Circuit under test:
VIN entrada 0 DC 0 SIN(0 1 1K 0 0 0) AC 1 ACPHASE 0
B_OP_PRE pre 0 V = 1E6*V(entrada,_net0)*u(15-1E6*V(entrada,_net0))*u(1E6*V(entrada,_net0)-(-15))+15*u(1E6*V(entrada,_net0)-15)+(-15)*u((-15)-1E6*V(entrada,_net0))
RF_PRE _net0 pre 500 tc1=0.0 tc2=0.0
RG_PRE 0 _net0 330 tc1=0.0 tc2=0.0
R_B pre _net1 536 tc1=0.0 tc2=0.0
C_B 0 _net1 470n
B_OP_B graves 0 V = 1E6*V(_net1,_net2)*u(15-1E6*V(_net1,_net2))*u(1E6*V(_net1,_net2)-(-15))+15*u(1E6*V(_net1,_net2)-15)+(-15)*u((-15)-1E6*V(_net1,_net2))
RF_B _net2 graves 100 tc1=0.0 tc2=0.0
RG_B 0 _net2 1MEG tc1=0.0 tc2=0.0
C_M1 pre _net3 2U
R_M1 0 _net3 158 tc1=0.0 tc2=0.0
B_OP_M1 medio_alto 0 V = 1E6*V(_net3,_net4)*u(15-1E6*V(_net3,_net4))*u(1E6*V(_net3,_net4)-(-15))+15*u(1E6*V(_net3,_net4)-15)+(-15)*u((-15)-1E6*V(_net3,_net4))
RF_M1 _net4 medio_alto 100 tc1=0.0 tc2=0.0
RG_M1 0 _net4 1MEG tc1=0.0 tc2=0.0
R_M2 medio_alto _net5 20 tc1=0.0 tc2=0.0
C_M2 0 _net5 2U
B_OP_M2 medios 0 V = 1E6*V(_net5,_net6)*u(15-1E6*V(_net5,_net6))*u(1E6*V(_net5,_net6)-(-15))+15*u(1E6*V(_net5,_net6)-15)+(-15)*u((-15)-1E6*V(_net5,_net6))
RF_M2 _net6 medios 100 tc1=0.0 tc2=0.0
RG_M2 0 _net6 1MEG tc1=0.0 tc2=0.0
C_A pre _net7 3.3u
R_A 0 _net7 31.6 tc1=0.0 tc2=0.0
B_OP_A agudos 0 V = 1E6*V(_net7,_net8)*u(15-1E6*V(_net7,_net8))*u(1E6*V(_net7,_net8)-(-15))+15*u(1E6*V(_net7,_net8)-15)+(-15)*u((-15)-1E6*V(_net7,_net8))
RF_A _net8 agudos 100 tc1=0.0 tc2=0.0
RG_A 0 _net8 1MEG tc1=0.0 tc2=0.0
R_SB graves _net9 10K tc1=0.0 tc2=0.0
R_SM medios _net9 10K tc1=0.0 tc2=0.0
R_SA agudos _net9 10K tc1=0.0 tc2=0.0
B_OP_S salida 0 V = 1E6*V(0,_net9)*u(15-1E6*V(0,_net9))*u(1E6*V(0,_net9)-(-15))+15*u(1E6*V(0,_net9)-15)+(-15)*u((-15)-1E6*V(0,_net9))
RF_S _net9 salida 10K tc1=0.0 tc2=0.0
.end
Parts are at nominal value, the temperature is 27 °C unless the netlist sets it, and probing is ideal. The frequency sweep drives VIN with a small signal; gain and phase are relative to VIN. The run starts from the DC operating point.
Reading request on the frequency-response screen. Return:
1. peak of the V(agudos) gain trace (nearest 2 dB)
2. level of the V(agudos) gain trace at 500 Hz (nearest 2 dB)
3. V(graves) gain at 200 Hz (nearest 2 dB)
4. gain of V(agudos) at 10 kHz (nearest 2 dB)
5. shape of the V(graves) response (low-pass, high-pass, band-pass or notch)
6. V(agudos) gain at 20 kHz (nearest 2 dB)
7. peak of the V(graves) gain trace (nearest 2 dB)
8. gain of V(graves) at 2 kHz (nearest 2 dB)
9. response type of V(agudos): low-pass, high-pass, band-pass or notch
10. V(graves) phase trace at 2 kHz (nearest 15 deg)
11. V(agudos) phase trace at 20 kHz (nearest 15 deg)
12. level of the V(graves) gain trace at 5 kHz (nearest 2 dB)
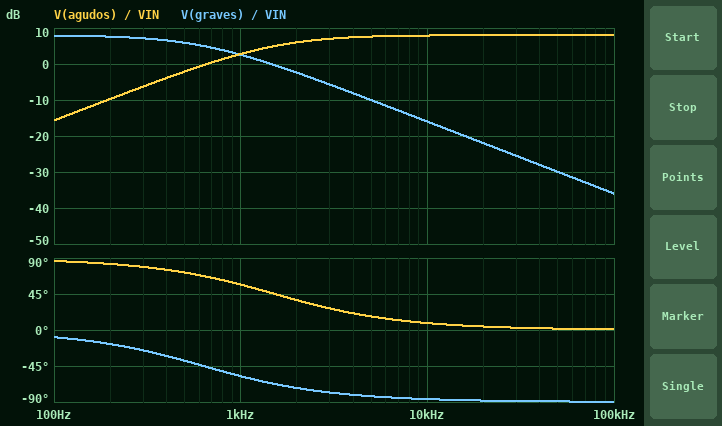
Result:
8 dB
-2 dB
8 dB
8 dB
low-pass
8 dB
8 dB
-2 dB
high-pass
-75 deg
0 deg
-10 dB
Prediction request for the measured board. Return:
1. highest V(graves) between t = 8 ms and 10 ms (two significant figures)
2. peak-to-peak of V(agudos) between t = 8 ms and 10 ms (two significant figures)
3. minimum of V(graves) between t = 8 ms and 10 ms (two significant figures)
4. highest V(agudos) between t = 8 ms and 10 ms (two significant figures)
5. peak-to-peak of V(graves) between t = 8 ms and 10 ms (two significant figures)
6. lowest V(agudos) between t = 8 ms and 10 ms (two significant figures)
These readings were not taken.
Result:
1.3 V
2.8 V
-1.3 V
1.4 V
2.7 V
-1.4 V
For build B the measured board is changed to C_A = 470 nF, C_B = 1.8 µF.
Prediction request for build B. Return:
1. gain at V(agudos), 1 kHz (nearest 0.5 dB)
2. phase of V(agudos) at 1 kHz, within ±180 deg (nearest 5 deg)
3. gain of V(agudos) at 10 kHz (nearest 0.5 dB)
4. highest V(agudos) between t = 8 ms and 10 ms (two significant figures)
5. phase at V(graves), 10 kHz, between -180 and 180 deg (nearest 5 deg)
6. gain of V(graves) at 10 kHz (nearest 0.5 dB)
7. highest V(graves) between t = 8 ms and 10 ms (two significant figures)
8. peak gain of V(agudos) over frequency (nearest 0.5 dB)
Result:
-12.5 dB
85 deg
4.5 dB
230 mV
-90 deg
-27.5 dB
410 mV
8.0 dB
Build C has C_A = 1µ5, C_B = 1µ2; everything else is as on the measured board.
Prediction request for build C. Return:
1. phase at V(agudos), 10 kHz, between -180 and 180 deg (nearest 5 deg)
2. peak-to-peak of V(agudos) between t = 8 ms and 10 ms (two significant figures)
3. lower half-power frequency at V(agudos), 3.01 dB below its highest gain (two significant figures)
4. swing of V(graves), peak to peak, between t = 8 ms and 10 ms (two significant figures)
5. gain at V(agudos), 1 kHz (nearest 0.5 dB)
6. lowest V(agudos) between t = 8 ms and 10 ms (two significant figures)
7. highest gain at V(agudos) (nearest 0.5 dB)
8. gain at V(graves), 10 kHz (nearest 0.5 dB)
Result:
20 deg
1.4 V
3.4 kHz
1.2 V
-3.0 dB
-720 mV
8.0 dB
-24.0 dB
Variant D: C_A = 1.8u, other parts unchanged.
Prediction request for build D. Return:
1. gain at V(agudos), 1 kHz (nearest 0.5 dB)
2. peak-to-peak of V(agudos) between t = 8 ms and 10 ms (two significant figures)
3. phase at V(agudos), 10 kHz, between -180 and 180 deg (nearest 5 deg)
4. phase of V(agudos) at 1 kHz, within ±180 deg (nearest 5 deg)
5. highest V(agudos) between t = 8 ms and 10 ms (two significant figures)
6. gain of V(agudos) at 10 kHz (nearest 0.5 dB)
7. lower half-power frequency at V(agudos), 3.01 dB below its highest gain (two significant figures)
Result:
-1.5 dB
1.7 V
15 deg
70 deg
850 mV
7.5 dB
2.8 kHz
